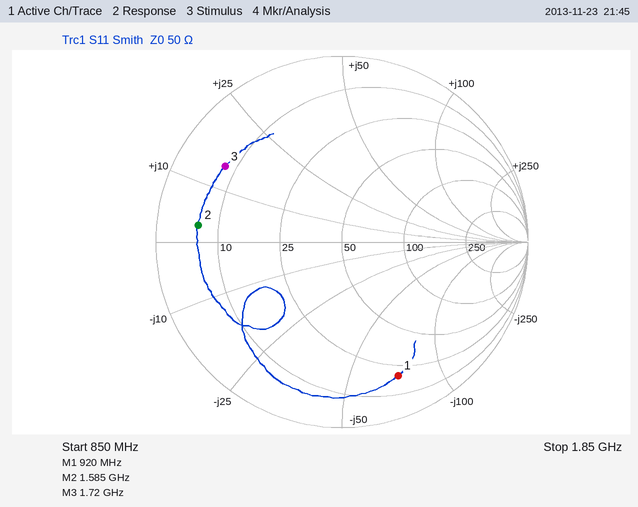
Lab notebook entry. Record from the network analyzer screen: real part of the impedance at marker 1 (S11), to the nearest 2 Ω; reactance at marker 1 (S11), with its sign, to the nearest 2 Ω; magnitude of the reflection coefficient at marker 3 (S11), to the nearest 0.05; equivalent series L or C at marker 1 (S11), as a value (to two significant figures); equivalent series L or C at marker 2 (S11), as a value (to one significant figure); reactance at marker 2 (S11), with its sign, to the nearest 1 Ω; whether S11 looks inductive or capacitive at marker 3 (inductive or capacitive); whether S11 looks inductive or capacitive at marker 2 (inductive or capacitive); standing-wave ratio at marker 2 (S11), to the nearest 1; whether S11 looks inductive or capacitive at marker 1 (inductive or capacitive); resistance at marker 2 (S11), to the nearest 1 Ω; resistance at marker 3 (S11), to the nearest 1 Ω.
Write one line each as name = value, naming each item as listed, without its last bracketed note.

real part of the impedance at marker 1 (S11), to the nearest 2 Ω = 20 Ω
reactance at marker 1 (S11), with its sign, to the nearest 2 Ω = -72 Ω
magnitude of the reflection coefficient at marker 3 (S11), to the nearest 0.05 = 0.75
equivalent series L or C at marker 1 (S11), as a value = 2.4 pF
equivalent series L or C at marker 2 (S11), as a value = 300 pH
reactance at marker 2 (S11), with its sign, to the nearest 1 Ω = +3 Ω
whether S11 looks inductive or capacitive at marker 3 = inductive
whether S11 looks inductive or capacitive at marker 2 = inductive
standing-wave ratio at marker 2 (S11), to the nearest 1 = 8
whether S11 looks inductive or capacitive at marker 1 = capacitive
resistance at marker 2 (S11), to the nearest 1 Ω = 6 Ω
resistance at marker 3 (S11), to the nearest 1 Ω = 8 Ω
